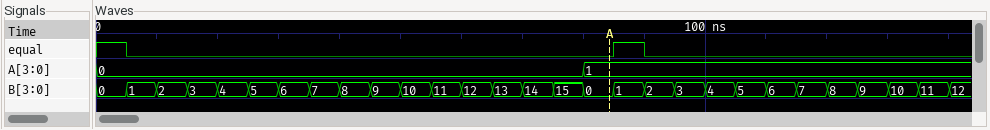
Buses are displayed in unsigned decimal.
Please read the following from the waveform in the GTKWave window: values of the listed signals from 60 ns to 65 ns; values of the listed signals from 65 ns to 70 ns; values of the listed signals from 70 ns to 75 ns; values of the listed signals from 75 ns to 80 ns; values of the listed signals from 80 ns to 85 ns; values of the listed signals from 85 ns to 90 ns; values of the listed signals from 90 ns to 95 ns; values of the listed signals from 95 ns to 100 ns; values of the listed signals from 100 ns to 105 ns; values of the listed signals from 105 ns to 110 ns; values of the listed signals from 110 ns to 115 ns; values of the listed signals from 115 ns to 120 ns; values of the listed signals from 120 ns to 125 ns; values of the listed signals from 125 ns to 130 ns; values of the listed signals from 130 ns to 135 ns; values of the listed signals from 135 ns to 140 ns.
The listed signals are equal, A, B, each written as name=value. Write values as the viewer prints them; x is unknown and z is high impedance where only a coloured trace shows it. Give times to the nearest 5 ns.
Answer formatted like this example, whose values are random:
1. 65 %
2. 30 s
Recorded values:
1. equal=0, A=0, B=12
2. equal=0, A=0, B=13
3. equal=0, A=0, B=14
4. equal=0, A=0, B=15
5. equal=0, A=1, B=0
6. equal=1, A=1, B=1
7. equal=0, A=1, B=2
8. equal=0, A=1, B=3
9. equal=0, A=1, B=4
10. equal=0, A=1, B=5
11. equal=0, A=1, B=6
12. equal=0, A=1, B=7
13. equal=0, A=1, B=8
14. equal=0, A=1, B=9
15. equal=0, A=1, B=10
16. equal=0, A=1, B=11
